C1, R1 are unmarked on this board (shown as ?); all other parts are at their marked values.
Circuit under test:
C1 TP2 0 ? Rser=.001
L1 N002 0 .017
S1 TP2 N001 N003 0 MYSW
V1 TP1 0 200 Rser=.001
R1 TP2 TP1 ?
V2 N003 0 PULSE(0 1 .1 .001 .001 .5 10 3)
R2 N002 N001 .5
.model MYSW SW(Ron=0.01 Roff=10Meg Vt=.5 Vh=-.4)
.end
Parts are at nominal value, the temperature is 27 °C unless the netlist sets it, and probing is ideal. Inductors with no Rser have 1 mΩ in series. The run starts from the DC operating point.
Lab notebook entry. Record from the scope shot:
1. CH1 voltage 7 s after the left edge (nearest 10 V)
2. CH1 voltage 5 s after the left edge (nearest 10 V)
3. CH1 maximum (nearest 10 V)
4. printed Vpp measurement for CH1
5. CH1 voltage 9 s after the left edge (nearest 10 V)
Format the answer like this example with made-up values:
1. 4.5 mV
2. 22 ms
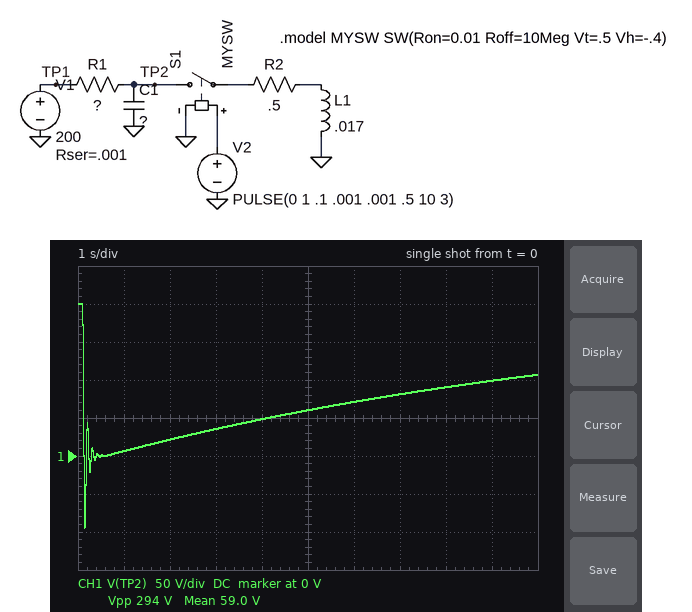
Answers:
1. 80 V
2. 60 V
3. 200 V
4. 294 V
5. 100 V
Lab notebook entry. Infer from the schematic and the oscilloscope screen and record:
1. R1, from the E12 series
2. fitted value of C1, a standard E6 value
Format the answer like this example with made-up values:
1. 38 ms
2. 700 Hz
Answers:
1. 820 Ω
2. 15 mF
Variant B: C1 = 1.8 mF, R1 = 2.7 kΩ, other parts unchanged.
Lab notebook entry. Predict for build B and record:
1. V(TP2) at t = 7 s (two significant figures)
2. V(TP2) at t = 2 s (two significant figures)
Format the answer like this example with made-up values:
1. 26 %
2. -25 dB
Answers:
1. 150 V
2. 50 V
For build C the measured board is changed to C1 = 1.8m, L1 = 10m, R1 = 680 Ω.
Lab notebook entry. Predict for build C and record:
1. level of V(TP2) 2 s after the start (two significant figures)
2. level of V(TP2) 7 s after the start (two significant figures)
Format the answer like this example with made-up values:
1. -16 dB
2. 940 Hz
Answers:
1. 140 V
2. 200 V
